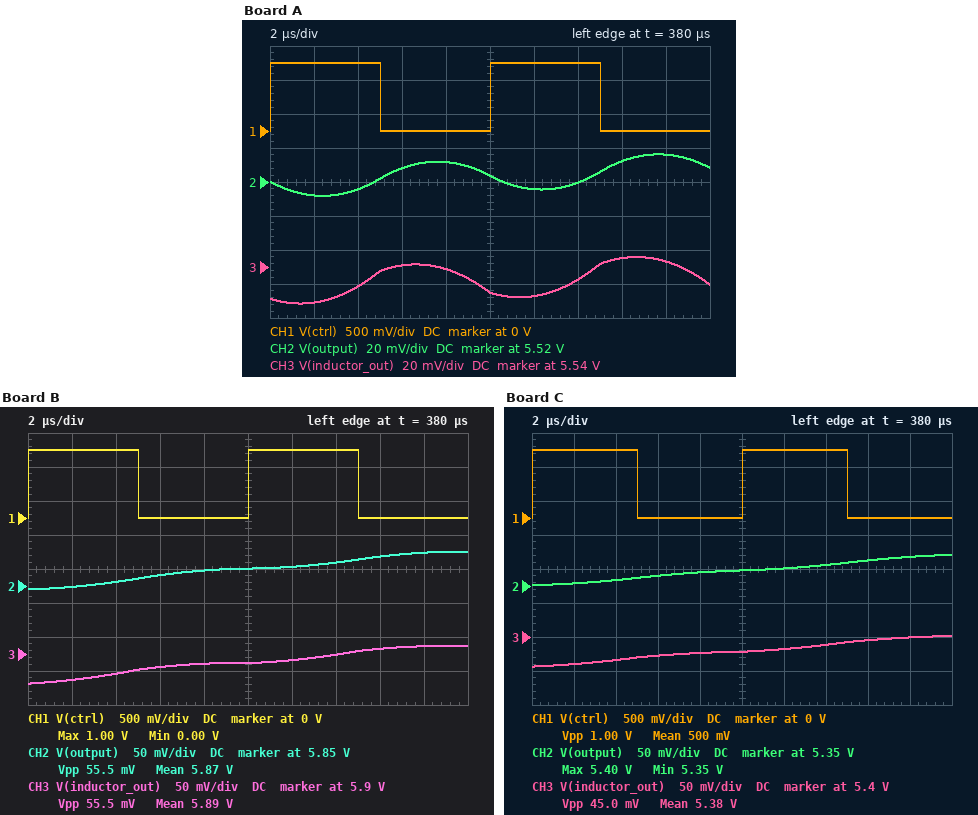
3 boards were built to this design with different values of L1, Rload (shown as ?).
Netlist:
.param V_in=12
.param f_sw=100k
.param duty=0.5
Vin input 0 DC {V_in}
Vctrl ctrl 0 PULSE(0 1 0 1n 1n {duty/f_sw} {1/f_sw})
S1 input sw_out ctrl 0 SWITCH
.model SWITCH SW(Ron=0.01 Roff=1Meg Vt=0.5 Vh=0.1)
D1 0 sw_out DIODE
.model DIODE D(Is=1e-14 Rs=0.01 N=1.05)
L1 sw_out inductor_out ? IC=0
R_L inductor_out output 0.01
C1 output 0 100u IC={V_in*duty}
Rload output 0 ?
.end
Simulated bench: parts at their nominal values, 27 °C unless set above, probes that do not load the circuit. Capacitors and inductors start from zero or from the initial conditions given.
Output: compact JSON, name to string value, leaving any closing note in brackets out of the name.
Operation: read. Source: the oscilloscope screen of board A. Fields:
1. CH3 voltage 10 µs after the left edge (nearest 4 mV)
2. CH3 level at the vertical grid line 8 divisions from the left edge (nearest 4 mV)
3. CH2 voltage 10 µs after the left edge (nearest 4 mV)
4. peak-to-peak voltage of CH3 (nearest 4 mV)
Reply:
{"CH3 voltage 10 µs after the left edge": "5.524 V", "CH3 level at the vertical grid line 8 divisions from the left edge": "5.544 V", "CH2 voltage 10 µs after the left edge": "5.524 V", "peak-to-peak voltage of CH3": "28 mV"}
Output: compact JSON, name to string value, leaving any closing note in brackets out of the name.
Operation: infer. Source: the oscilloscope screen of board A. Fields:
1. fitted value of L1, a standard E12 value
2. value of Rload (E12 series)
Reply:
{"fitted value of L1, a standard E12 value": "22 µH", "value of Rload": "6.8 Ω"}
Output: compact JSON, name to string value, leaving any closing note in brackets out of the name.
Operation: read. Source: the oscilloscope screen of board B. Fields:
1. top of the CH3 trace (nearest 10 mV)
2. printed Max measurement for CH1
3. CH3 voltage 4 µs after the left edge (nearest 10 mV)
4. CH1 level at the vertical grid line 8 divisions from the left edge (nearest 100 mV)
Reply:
{"top of the CH3 trace": "5.91 V", "printed Max measurement for CH1": "1.00 V", "CH3 voltage 4 µs after the left edge": "5.87 V", "CH1 level at the vertical grid line 8 divisions from the left edge": "0 V"}
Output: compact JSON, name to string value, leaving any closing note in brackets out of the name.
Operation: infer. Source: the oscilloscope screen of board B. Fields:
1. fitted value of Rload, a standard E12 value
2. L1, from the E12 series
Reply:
{"fitted value of Rload, a standard E12 value": "5.6 Ω", "L1, from the E12 series": "68 µH"}
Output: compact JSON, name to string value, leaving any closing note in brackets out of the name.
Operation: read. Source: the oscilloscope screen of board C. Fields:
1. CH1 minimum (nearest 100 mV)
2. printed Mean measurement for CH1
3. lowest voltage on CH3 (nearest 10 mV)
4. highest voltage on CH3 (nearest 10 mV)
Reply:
{"CH1 minimum": "0 V", "printed Mean measurement for CH1": "500 mV", "lowest voltage on CH3": "5.36 V", "highest voltage on CH3": "5.40 V"}
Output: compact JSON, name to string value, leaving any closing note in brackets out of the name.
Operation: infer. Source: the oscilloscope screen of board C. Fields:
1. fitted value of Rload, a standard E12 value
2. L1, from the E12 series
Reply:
{"fitted value of Rload, a standard E12 value": "12 Ω", "L1, from the E12 series": "120 µH"}
